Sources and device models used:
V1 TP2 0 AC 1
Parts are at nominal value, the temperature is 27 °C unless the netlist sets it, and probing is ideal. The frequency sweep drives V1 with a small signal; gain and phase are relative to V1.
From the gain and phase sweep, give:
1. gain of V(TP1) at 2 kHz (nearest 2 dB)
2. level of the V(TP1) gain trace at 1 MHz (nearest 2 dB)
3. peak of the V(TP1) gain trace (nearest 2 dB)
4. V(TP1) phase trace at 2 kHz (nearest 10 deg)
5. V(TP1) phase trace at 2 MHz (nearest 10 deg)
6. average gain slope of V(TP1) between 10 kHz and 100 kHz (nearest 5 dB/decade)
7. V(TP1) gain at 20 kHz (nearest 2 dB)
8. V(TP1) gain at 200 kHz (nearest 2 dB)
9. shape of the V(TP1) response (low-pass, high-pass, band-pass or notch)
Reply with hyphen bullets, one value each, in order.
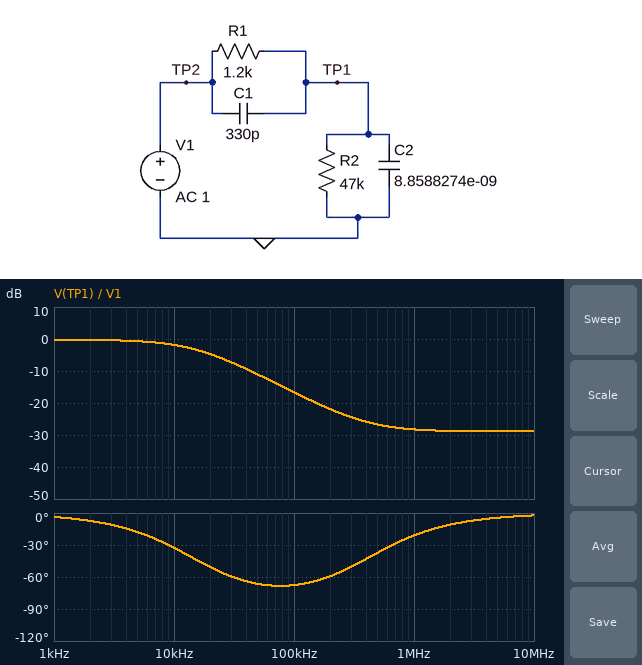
- 0 dB
- -28 dB
- 0 dB
- -10 deg
- -10 deg
- -15 dB/decade
- -4 dB
- -22 dB
- low-pass
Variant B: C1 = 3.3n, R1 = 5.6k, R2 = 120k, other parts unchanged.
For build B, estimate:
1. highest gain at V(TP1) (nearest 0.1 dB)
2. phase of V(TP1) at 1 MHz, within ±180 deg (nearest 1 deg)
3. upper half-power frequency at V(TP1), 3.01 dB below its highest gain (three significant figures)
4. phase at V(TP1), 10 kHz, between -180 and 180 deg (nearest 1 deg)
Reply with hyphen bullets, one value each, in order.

- -0.4 dB
- 0 deg
- 2.67 kHz
- -27 deg
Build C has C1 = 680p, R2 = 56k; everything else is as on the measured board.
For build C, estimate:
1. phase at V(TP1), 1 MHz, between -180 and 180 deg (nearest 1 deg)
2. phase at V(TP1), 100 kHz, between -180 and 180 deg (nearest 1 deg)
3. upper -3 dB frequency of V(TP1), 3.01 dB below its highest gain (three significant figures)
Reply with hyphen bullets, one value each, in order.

- -10 deg
- -55 deg
- 14.3 kHz
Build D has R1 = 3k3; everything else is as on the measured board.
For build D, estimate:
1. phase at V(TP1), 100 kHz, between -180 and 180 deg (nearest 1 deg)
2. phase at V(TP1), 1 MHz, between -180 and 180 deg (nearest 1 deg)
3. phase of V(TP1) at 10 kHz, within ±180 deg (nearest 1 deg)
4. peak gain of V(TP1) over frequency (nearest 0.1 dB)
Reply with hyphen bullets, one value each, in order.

- -52 deg
- -8 deg
- -57 deg
- -0.6 dB
